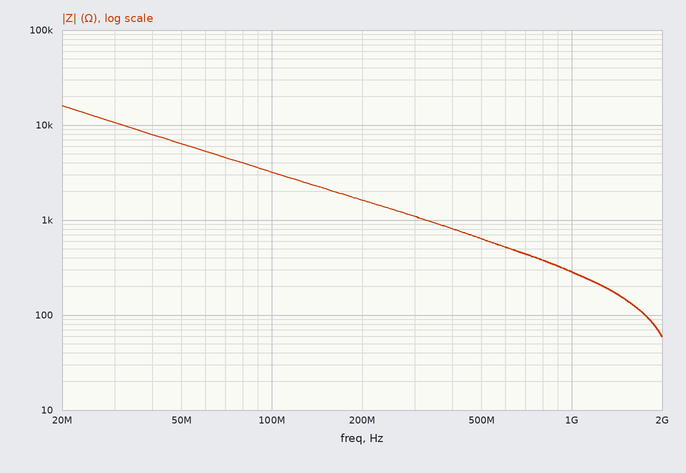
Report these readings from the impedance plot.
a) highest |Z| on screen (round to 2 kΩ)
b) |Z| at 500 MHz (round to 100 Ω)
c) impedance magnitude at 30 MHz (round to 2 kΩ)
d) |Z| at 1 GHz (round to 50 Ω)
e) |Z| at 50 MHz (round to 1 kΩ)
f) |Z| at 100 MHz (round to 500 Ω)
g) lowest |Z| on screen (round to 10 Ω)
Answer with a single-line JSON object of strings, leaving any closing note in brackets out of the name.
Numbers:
{"highest |Z| on screen": "16 kΩ", "|Z| at 500 MHz": "600 Ω", "impedance magnitude at 30 MHz": "10 kΩ", "|Z| at 1 GHz": "300 Ω", "|Z| at 50 MHz": "6 kΩ", "|Z| at 100 MHz": "3.0 kΩ", "lowest |Z| on screen": "60 Ω"}
